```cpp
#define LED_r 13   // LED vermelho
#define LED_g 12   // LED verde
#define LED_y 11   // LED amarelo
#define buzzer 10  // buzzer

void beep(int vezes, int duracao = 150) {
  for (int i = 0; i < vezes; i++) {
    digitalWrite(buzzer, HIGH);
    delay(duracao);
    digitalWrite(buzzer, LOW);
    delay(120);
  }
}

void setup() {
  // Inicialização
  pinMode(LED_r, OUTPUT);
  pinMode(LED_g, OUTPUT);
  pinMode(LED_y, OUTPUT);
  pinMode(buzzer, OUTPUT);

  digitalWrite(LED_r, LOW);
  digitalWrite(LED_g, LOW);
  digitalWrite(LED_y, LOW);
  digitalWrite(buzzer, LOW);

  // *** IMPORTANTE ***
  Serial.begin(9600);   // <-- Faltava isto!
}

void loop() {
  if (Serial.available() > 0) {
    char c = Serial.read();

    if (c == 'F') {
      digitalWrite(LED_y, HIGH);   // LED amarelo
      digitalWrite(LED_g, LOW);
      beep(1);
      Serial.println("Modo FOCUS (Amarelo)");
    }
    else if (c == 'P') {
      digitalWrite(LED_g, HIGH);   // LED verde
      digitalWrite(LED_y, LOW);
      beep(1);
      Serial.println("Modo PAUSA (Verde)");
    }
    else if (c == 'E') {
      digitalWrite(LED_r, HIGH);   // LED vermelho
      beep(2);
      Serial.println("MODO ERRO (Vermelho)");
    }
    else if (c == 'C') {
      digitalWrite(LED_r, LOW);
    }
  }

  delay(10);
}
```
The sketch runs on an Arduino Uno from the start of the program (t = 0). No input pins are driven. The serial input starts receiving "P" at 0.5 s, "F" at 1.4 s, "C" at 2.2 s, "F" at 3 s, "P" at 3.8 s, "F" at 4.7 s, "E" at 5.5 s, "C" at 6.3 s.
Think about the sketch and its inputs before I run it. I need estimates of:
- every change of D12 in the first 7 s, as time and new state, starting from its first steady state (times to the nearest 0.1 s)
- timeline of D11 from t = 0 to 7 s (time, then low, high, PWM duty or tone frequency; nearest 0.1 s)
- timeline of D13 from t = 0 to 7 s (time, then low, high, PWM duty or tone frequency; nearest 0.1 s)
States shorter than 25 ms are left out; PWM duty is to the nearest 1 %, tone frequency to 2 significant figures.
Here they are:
0 s low; 0.5 s high; 1.4 s low; 3.8 s high; 4.7 s low
0 s low; 1.4 s high; 3.8 s low; 4.7 s high
0 s low; 5.5 s high; 6.3 s low
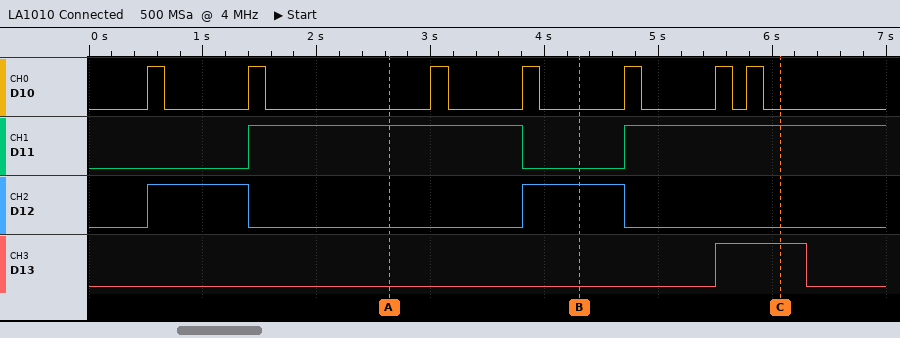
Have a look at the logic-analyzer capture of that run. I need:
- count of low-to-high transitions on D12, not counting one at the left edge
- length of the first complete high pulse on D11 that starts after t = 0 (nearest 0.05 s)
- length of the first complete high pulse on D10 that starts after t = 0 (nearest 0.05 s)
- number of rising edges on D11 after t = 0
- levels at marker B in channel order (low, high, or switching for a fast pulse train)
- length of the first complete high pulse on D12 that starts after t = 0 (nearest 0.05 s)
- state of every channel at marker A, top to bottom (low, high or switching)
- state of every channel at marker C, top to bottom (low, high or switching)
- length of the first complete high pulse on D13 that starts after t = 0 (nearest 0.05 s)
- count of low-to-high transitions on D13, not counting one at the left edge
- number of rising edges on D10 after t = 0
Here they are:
2
2.40 s
0.15 s
2
D10 low, D11 low, D12 high, D13 low
0.90 s
D10 low, D11 high, D12 low, D13 low
D10 low, D11 high, D12 low, D13 high
0.80 s
1
7
